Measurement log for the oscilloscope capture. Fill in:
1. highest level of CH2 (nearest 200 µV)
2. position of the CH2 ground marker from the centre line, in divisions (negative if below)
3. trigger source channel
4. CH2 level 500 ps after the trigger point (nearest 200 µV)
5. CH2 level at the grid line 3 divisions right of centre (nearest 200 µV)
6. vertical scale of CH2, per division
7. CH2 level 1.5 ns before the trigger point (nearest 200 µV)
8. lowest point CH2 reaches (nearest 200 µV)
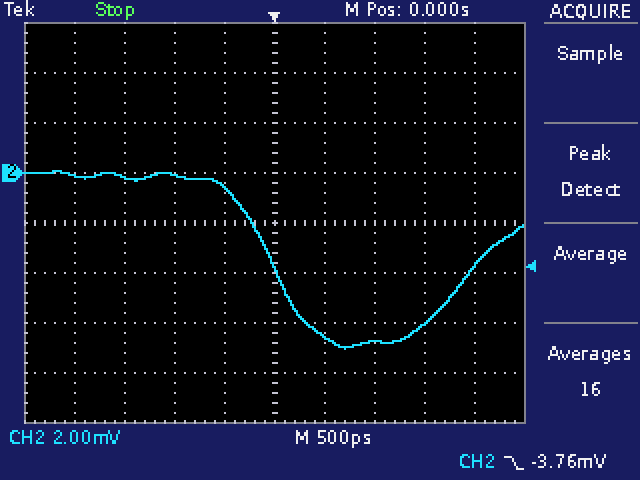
0.0 mV
+1.0 div
CH2
-6.6 mV
-6.0 mV
2 mV
-200 µV
-7.0 mV
